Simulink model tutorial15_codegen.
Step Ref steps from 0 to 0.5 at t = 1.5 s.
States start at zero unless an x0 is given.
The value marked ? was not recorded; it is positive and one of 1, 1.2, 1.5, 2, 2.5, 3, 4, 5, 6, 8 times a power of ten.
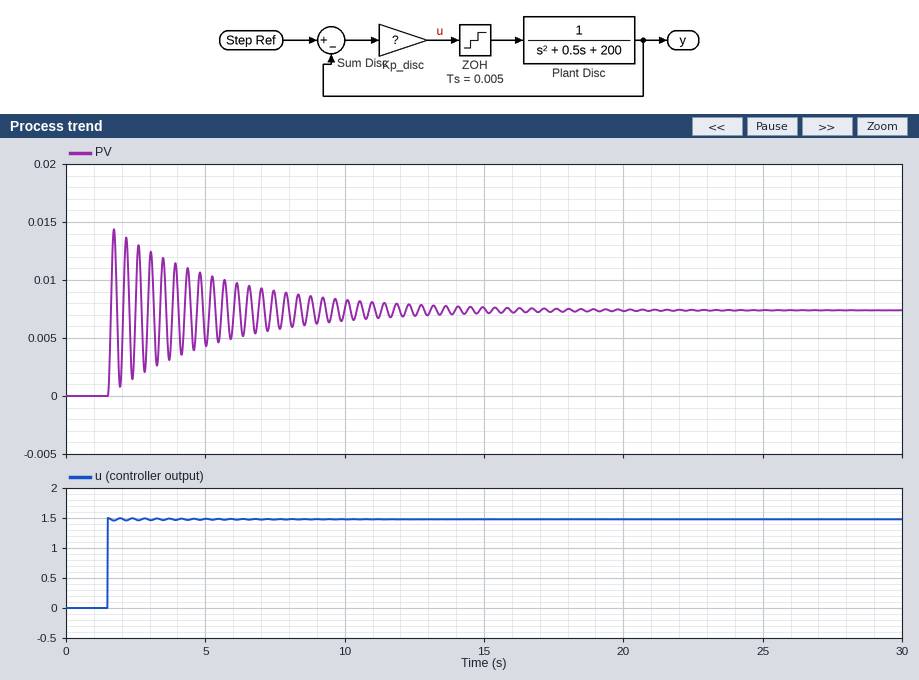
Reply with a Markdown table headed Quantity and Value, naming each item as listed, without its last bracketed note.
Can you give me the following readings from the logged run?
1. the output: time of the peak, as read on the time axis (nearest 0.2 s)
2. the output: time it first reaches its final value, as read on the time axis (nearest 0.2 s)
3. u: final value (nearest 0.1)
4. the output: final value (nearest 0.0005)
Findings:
| Quantity | Value |
|---|---|
| the output: time of the peak, as read on the time axis | 1.8 s |
| the output: time it first reaches its final value, as read on the time axis | 1.6 s |
| u: final value | 1.5 |
| the output: final value | 0.0075 |
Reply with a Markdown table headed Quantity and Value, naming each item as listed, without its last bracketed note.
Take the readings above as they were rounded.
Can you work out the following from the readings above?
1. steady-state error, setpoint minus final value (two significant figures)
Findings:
| Quantity | Value |
|---|---|
| steady-state error, setpoint minus final value | 0.49 |
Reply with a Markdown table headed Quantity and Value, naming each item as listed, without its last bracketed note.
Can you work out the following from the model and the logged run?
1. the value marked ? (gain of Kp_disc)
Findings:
| Quantity | Value |
|---|---|
| the value marked ? | 3 |
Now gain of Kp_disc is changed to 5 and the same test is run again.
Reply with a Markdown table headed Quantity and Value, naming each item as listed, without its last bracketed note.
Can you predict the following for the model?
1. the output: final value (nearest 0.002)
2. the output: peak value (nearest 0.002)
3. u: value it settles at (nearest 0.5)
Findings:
| Quantity | Value |
|---|---|
| the output: final value | 0.012 |
| the output: peak value | 0.024 |
| u: value it settles at | 2.5 |
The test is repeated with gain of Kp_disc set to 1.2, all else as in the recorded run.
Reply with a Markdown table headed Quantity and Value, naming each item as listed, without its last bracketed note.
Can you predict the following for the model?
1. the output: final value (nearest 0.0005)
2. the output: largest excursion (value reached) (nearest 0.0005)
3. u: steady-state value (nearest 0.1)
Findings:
| Quantity | Value |
|---|---|
| the output: final value | 0.0030 |
| the output: largest excursion (value reached) | 0.0060 |
| u: steady-state value | 0.6 |
